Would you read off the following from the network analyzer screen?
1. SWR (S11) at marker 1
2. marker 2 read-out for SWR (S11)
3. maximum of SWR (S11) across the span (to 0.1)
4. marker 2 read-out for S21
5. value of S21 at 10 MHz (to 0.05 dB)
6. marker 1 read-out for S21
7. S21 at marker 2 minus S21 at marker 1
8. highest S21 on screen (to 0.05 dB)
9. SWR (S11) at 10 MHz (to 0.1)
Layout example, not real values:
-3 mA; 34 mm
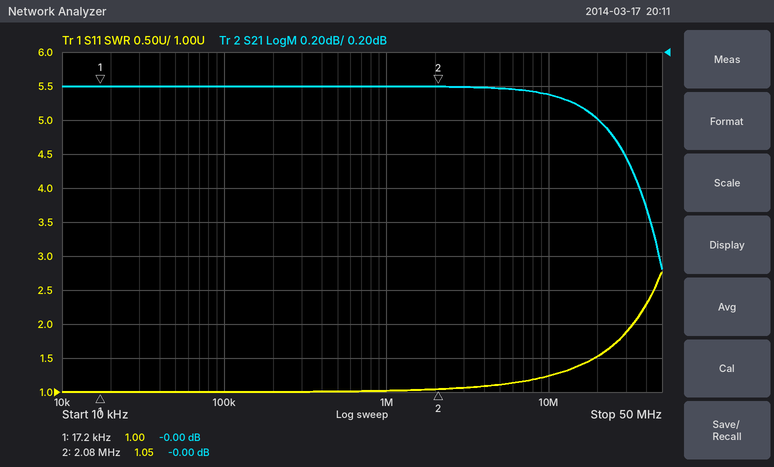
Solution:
1.00; 1.05; 2.8; -0.00 dB; -0.05 dB; -0.00 dB; 0.00 dB; 0.00 dB; 1.2
